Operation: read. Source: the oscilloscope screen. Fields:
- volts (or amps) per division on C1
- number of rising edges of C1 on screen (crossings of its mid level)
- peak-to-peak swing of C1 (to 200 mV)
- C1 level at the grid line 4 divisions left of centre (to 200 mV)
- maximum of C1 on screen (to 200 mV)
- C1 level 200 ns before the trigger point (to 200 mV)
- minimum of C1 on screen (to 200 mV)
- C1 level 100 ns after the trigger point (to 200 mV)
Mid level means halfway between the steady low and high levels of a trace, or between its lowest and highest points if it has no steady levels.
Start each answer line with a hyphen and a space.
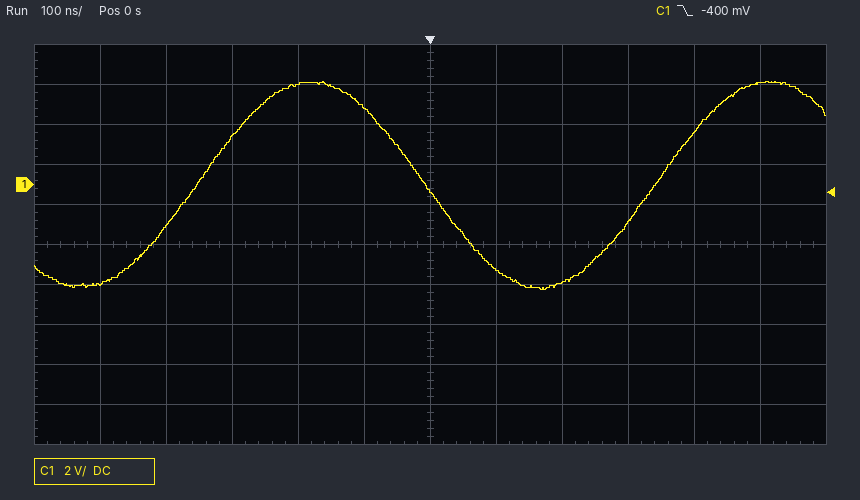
- 2 V
- 2
- 10.4 V
- -2.0 V
- 5.2 V
- 5.0 V
- -5.2 V
- -4.2 V
